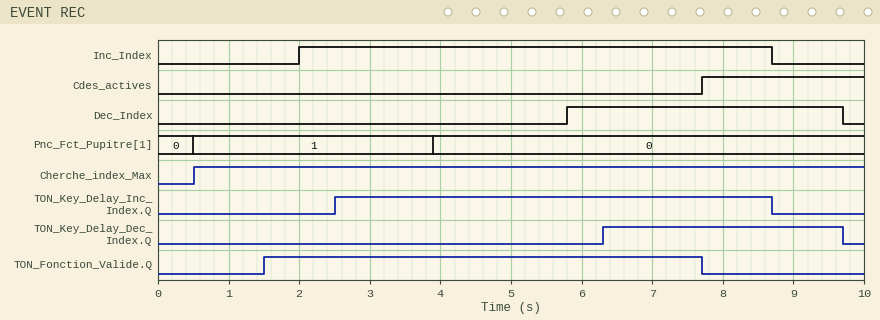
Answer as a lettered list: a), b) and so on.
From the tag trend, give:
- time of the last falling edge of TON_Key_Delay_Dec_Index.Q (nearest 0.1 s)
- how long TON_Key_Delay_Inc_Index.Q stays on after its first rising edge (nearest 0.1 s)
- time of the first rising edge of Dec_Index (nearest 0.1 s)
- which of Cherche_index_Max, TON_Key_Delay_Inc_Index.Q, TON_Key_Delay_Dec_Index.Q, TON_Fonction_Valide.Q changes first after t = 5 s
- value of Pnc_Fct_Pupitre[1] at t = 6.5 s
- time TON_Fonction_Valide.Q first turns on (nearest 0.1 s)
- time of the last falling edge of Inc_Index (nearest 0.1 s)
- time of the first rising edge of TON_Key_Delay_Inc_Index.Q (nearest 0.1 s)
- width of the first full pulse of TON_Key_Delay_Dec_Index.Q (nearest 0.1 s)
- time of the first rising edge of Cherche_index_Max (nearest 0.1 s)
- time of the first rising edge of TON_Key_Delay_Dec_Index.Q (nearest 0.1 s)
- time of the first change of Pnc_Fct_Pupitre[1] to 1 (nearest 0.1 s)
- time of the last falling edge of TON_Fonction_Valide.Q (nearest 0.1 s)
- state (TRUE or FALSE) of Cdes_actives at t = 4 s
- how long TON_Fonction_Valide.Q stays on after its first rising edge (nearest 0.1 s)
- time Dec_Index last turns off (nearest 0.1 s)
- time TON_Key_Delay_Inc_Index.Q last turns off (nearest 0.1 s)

a) 9.7 s
b) 6.2 s
c) 5.8 s
d) TON_Key_Delay_Dec_Index.Q
e) 0
f) 1.5 s
g) 8.7 s
h) 2.5 s
i) 3.4 s
j) 0.5 s
k) 6.3 s
l) 0.5 s
m) 7.7 s
n) FALSE
o) 6.2 s
p) 9.7 s
q) 8.7 s
